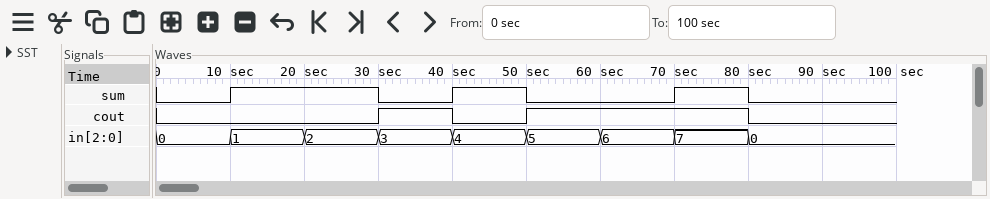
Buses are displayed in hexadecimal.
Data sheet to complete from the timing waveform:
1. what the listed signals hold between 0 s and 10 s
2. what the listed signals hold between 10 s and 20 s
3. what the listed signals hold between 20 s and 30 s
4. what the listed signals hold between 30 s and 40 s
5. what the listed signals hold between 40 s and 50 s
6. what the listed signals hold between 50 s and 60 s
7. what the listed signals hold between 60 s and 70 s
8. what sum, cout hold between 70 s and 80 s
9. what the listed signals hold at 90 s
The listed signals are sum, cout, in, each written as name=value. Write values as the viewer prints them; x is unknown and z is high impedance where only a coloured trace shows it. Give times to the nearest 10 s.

sum=0, cout=0, in=0
sum=1, cout=0, in=1
sum=1, cout=0, in=2
sum=0, cout=1, in=3
sum=1, cout=0, in=4
sum=0, cout=1, in=5
sum=0, cout=1, in=6
sum=1, cout=1
sum=0, cout=0, in=0
